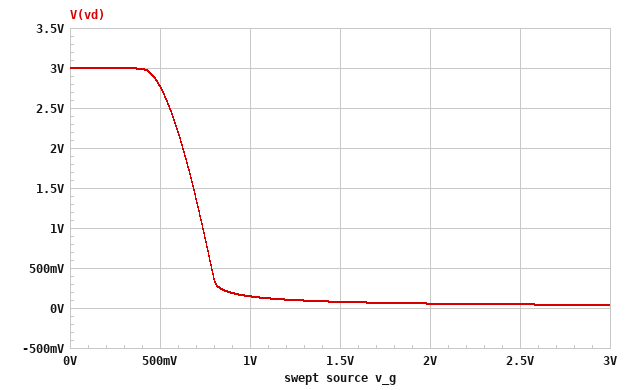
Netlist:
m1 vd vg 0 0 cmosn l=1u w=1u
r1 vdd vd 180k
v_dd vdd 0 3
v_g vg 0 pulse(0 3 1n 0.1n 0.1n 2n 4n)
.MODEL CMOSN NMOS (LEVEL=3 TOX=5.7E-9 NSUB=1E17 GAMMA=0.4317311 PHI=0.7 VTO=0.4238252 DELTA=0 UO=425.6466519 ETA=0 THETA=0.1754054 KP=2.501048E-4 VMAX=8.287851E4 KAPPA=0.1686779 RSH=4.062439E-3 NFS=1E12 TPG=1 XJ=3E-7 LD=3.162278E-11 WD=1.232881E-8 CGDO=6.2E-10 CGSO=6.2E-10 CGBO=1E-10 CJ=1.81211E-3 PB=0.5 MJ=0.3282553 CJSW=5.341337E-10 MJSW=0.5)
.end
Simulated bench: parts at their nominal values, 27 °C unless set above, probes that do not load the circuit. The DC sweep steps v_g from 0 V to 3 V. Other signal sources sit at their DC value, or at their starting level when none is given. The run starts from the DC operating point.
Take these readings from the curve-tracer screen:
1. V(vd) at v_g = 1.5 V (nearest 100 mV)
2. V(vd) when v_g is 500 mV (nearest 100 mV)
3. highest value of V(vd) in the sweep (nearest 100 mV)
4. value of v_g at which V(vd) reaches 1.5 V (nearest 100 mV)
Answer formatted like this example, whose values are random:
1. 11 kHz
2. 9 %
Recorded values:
1. 100 mV
2. 2.8 V
3. 3.0 V
4. 700 mV
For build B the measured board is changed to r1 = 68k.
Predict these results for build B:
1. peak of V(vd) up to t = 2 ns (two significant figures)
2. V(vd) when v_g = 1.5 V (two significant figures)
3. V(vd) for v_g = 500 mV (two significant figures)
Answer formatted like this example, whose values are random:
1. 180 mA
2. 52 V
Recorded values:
1. 3.5 V
2. 220 mV
3. 2.9 V
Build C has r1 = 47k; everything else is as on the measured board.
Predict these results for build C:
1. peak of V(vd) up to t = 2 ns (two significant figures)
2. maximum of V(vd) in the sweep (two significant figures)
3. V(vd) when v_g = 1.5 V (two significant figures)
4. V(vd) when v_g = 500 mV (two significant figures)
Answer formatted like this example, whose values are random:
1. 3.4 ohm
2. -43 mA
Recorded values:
1. 3.4 V
2. 3.0 V
3. 350 mV
4. 2.9 V
